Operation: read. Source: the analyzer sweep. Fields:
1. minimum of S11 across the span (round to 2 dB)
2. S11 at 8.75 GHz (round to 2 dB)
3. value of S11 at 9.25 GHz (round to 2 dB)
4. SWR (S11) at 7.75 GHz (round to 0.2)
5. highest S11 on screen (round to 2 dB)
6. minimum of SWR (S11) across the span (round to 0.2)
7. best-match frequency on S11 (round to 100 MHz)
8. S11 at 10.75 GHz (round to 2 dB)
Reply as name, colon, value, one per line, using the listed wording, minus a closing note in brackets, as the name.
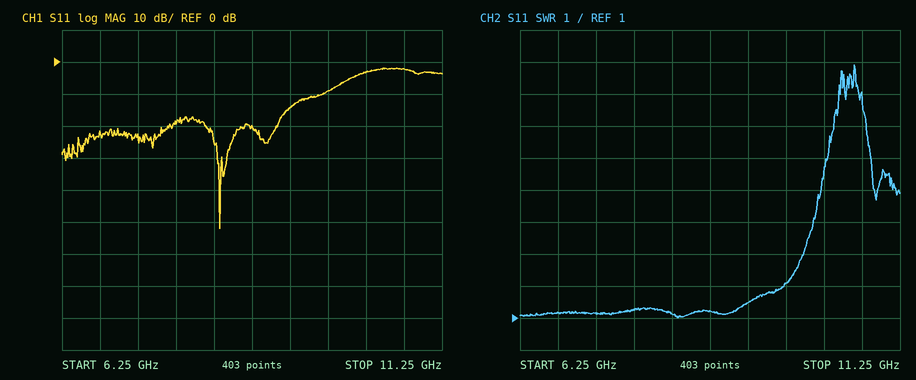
minimum of S11 across the span: -52 dB
S11 at 8.75 GHz: -20 dB
value of S11 at 9.25 GHz: -14 dB
SWR (S11) at 7.75 GHz: 1.2
highest S11 on screen: -2 dB
minimum of SWR (S11) across the span: 1.0
best-match frequency on S11: 8.3 GHz
S11 at 10.75 GHz: -2 dB
